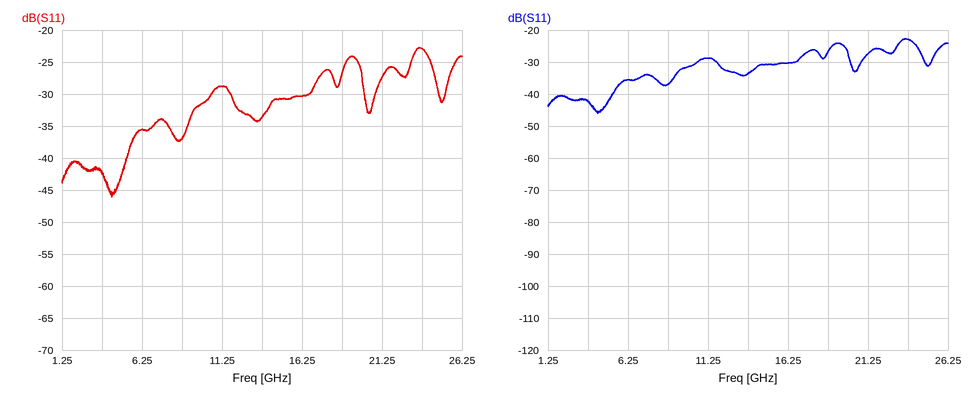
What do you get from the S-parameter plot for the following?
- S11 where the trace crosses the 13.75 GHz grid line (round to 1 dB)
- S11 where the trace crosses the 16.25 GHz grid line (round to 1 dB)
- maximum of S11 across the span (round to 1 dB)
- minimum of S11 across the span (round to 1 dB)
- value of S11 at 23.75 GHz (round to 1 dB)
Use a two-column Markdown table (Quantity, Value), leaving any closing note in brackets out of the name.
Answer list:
| Quantity | Value |
|---|---|
| S11 where the trace crosses the 13.75 GHz grid line | -34 dB |
| S11 where the trace crosses the 16.25 GHz grid line | -30 dB |
| maximum of S11 across the span | -23 dB |
| minimum of S11 across the span | -46 dB |
| value of S11 at 23.75 GHz | -23 dB |
